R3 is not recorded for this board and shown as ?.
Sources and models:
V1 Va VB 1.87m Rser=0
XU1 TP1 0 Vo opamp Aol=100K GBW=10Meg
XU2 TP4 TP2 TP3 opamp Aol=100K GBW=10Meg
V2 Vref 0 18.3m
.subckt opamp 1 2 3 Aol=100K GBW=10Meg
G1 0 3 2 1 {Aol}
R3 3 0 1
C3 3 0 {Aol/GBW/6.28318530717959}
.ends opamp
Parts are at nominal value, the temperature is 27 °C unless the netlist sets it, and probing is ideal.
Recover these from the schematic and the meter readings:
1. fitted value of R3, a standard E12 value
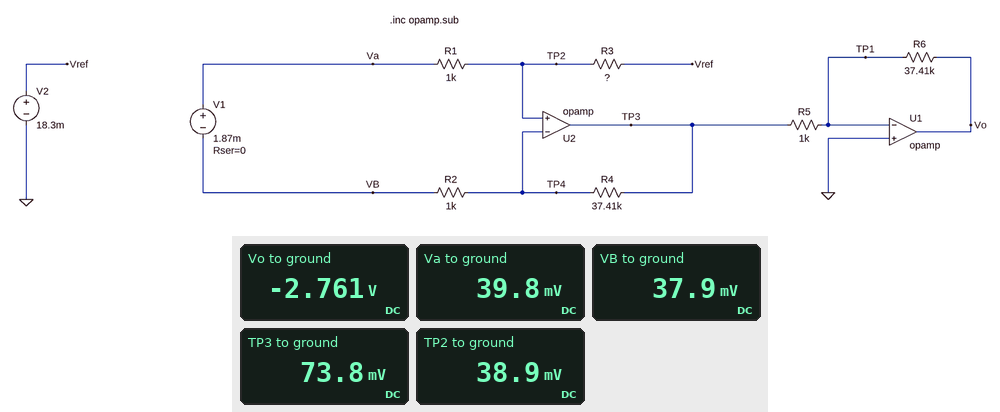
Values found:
22 kΩ
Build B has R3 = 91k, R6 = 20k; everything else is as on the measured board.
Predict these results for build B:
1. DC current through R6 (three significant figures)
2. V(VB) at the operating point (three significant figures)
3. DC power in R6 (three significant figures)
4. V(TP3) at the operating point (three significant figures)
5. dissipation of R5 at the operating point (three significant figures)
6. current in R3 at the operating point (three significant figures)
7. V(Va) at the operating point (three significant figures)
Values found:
138 µA
102 mV
382 µW
138 mV
19.1 µW
934 nA
104 mV
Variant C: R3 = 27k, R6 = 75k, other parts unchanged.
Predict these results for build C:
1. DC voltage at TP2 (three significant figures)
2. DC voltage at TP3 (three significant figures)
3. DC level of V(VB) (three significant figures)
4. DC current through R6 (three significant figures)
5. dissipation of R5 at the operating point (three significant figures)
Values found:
43.5 mV
78.5 mV
42.6 mV
78.4 µA
6.15 µW
